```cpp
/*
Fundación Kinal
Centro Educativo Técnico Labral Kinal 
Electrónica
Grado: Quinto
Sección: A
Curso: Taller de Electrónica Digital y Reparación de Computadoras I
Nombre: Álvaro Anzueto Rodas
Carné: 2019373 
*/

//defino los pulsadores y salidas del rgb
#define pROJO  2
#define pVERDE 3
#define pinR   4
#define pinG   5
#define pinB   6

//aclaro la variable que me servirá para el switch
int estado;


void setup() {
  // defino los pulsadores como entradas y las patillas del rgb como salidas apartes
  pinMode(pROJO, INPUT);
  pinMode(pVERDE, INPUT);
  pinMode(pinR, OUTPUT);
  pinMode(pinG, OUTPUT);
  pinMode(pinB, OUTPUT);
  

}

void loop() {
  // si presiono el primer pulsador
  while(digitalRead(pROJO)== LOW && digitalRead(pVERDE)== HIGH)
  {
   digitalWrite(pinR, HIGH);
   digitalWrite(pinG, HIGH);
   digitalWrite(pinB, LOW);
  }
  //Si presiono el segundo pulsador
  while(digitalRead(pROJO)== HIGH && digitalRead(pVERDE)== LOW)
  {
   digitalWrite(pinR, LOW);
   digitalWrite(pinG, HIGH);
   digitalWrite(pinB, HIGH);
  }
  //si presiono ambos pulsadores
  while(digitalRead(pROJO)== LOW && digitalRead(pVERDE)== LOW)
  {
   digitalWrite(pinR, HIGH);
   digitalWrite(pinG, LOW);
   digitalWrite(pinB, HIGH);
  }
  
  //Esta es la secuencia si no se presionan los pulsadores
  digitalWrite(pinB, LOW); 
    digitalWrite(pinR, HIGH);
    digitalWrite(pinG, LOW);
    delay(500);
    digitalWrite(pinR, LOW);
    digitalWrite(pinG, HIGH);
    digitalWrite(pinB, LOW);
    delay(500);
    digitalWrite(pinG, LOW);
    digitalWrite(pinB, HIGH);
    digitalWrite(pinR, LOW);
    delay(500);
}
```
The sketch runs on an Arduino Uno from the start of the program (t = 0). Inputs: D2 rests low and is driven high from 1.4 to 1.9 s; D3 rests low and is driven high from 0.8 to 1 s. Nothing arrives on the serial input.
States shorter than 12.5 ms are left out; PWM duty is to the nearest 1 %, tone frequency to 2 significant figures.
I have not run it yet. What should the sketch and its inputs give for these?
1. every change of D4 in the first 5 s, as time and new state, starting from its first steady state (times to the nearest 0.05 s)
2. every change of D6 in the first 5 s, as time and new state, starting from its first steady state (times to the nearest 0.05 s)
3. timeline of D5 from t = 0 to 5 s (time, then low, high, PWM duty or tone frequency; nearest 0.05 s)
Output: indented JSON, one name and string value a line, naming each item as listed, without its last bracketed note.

{
  "every change of D4 in the first 5 s, as time and new state, starting from its first steady state": "0 s high; 1.3 s low; 2.3 s high",
  "every change of D6 in the first 5 s, as time and new state, starting from its first steady state": "0 s high; 0.8 s low; 1.8 s high",
  "timeline of D5 from t = 0 to 5 s": "0 s low; 1.3 s high; 1.8 s low"
}
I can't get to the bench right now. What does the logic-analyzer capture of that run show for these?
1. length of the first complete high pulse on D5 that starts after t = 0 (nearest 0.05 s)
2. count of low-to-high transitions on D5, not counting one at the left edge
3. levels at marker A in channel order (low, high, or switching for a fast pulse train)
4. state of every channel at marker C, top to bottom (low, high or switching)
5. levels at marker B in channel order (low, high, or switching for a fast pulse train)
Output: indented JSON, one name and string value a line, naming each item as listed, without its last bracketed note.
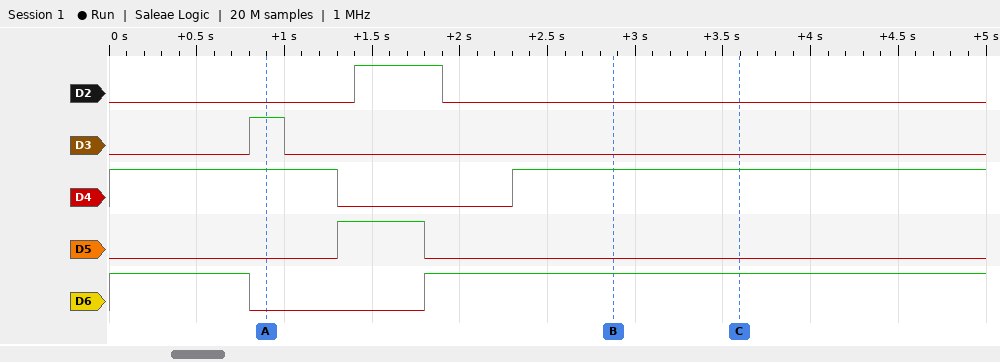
{
  "length of the first complete high pulse on D5 that starts after t = 0": "0.50 s",
  "count of low-to-high transitions on D5, not counting one at the left edge": "1",
  "levels at marker A in channel order": "D2 low, D3 high, D4 high, D5 low, D6 low",
  "state of every channel at marker C, top to bottom": "D2 low, D3 low, D4 high, D5 low, D6 high",
  "levels at marker B in channel order": "D2 low, D3 low, D4 high, D5 low, D6 high"
}
